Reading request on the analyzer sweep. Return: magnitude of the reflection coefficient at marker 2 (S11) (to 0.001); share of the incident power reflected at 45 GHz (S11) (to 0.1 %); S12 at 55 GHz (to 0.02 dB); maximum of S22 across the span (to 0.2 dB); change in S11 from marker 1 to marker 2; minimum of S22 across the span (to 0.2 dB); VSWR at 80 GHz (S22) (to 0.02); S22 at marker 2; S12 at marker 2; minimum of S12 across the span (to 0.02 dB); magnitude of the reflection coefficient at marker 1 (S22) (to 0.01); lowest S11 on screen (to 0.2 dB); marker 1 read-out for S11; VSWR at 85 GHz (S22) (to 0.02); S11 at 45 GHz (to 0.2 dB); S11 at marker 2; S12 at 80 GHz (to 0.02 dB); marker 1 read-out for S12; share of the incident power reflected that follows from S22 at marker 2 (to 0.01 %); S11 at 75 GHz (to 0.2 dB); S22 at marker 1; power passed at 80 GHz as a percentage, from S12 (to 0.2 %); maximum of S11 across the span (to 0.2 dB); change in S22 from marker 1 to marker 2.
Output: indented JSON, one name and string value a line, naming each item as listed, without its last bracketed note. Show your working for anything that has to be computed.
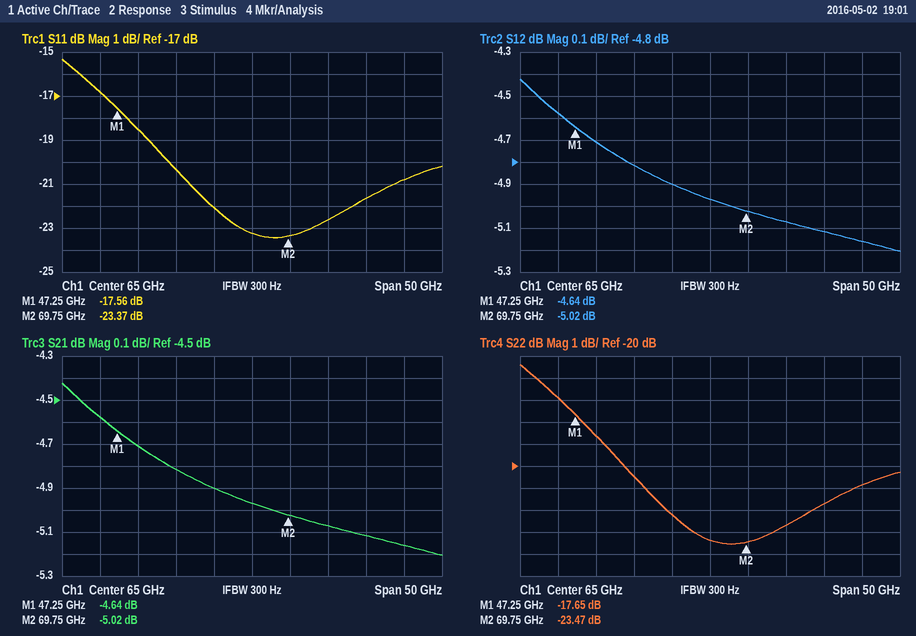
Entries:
{
  "magnitude of the reflection coefficient at marker 2 (S11)": "10^(-23.37/20) ≈ 0.068",
  "share of the incident power reflected at 45 GHz (S11)": "10^(-16.8/10) ≈ 2.1 %",
  "S12 at 55 GHz": "-4.82 dB",
  "maximum of S22 across the span": "-15.4 dB",
  "change in S11 from marker 1 to marker 2": "-23.37 − (-17.56) = -5.81 dB",
  "minimum of S22 across the span": "-23.6 dB",
  "VSWR at 80 GHz (S22)": "|Γ| = 10^(-21.8/20) = 0.0813; VSWR = (1 + 0.0813)/(1 − 0.0813) ≈ 1.18",
  "S22 at marker 2": "-23.47 dB",
  "S12 at marker 2": "-5.02 dB",
  "minimum of S12 across the span": "-5.20 dB",
  "magnitude of the reflection coefficient at marker 1 (S22)": "10^(-17.65/20) ≈ 0.13",
  "lowest S11 on screen": "-23.4 dB",
  "marker 1 read-out for S11": "-17.56 dB",
  "VSWR at 85 GHz (S22)": "|Γ| = 10^(-20.8/20) = 0.0912; VSWR = (1 + 0.0912)/(1 − 0.0912) ≈ 1.20",
  "S11 at 45 GHz": "-16.8 dB",
  "S11 at marker 2": "-23.37 dB",
  "S12 at 80 GHz": "-5.12 dB",
  "marker 1 read-out for S12": "-4.64 dB",
  "share of the incident power reflected that follows from S22 at marker 2": "10^(-23.47/10) ≈ 0.45 %",
  "S11 at 75 GHz": "-22.6 dB",
  "S22 at marker 1": "-17.65 dB",
  "power passed at 80 GHz as a percentage, from S12": "10^(-5.12/10) ≈ 30.8 %",
  "maximum of S11 across the span": "-15.4 dB",
  "change in S22 from marker 1 to marker 2": "-23.47 − (-17.65) = -5.82 dB"
}
